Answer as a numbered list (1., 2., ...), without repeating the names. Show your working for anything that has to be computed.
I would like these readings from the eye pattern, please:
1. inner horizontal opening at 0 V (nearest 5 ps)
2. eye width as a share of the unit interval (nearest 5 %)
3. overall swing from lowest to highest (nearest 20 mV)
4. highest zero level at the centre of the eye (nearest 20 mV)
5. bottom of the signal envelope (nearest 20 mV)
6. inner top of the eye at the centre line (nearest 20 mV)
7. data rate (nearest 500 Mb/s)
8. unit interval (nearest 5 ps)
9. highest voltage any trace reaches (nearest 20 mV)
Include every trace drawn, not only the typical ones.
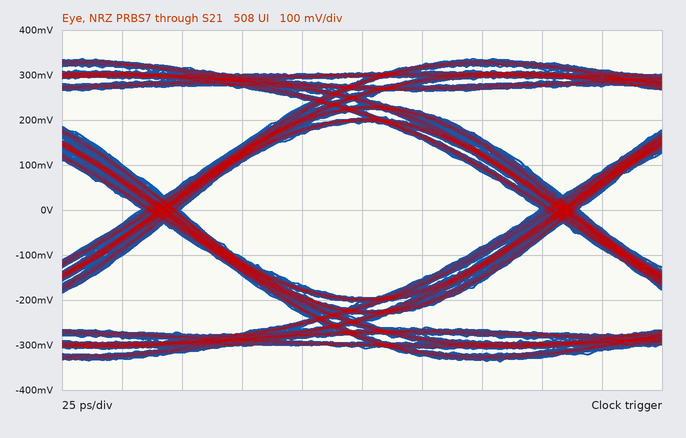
1. 150 ps
2. 150 ps / 165 ps ≈ 90.9 %, so 90 % to the nearest 5 %
3. 680 mV
4. -200 mV
5. -340 mV
6. 200 mV
7. 6.0 Gb/s
8. 165 ps
9. 340 mV
